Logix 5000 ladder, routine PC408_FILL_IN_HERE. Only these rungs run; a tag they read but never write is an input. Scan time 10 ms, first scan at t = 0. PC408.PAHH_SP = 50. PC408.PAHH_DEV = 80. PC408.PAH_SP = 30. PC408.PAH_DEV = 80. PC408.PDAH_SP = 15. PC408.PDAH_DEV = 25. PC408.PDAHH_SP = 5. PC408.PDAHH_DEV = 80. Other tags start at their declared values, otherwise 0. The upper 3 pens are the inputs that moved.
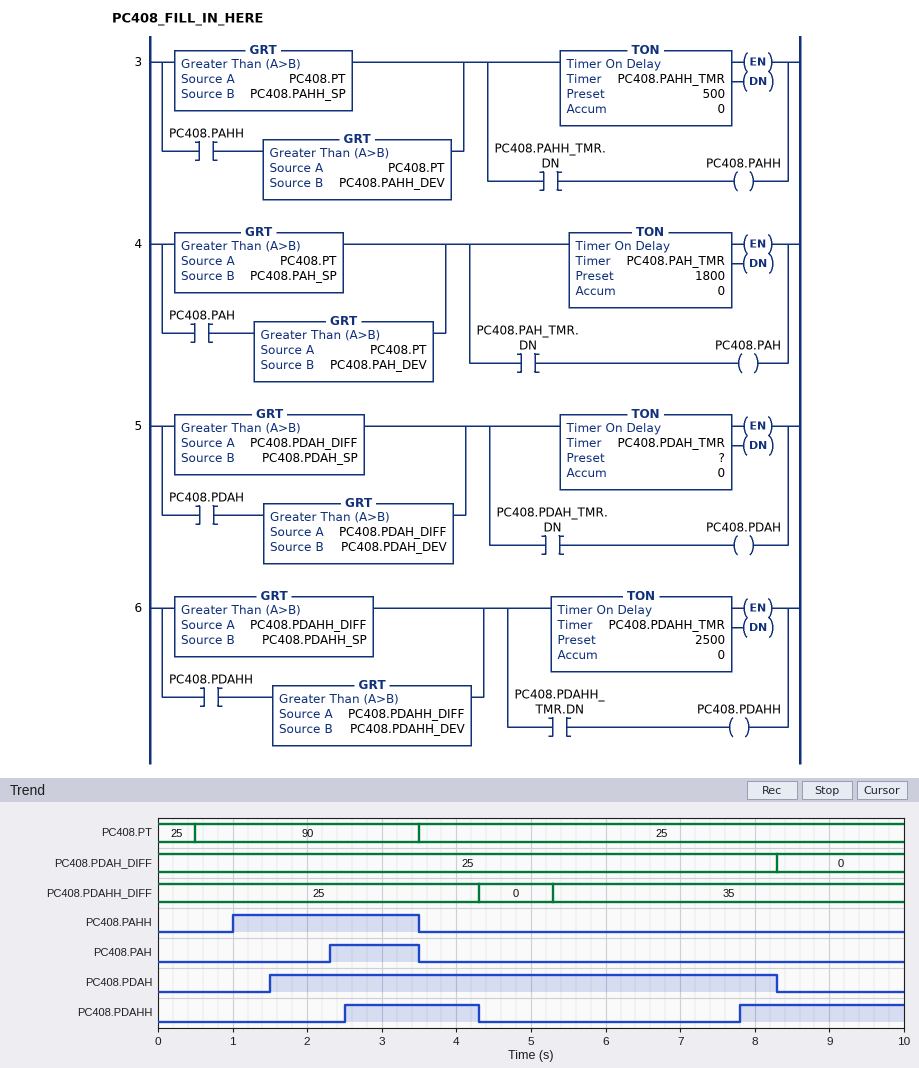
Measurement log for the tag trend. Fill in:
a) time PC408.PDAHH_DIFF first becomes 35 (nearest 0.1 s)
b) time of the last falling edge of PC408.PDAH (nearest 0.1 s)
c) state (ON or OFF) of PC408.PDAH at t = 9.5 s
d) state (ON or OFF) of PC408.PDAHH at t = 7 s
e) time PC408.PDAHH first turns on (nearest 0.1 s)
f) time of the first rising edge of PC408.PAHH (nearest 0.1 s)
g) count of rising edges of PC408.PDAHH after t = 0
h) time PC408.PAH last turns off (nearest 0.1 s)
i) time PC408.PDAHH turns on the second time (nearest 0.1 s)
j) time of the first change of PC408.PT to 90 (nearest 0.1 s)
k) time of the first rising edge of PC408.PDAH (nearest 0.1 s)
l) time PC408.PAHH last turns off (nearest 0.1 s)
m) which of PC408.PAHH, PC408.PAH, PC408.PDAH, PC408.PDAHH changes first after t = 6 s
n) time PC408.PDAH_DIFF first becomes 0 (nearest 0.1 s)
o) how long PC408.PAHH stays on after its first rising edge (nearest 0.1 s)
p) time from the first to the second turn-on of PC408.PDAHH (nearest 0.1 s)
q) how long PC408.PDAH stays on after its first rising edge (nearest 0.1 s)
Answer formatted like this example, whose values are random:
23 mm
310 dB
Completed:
5.3 s
8.3 s
OFF
OFF
2.5 s
1.0 s
2
3.5 s
7.8 s
0.5 s
1.5 s
3.5 s
PC408.PDAHH
8.3 s
2.5 s
5.3 s
6.8 s
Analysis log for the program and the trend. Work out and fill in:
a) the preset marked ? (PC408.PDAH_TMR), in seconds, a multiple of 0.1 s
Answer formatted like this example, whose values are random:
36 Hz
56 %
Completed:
1.5 s
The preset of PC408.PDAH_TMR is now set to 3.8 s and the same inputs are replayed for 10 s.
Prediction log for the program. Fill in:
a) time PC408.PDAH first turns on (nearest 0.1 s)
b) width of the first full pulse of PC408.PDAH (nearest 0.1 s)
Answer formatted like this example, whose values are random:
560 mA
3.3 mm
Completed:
3.8 s
4.5 s
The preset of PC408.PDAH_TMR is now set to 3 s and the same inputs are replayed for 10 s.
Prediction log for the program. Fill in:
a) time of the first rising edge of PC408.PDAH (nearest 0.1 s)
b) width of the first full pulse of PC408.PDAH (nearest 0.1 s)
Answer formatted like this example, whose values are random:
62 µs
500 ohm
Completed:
3.0 s
5.3 s
